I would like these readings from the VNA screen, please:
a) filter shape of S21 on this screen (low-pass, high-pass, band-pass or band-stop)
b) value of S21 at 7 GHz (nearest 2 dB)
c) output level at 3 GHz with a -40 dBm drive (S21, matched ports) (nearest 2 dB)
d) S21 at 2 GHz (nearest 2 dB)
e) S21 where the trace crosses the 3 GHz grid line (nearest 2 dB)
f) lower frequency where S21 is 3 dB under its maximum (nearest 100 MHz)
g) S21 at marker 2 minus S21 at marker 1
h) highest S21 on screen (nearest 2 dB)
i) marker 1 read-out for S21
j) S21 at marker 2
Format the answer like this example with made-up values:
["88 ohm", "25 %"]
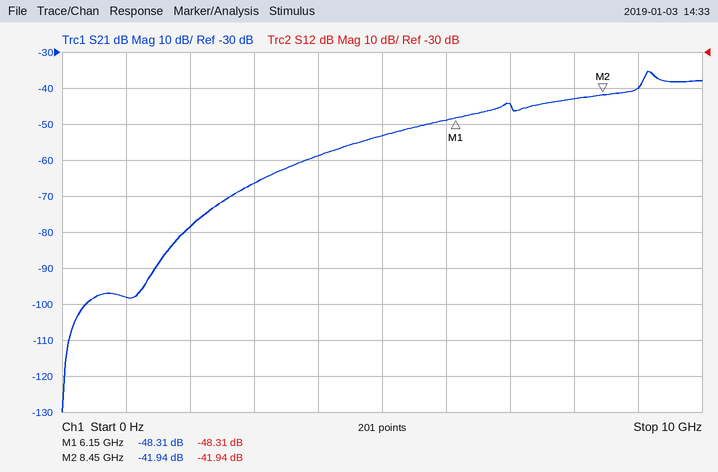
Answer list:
["high-pass", "-44 dB", "-106 dBm", "-78 dB", "-66 dB", "9.1 GHz", "6.37 dB", "-36 dB", "-48.31 dB", "-41.94 dB"]
